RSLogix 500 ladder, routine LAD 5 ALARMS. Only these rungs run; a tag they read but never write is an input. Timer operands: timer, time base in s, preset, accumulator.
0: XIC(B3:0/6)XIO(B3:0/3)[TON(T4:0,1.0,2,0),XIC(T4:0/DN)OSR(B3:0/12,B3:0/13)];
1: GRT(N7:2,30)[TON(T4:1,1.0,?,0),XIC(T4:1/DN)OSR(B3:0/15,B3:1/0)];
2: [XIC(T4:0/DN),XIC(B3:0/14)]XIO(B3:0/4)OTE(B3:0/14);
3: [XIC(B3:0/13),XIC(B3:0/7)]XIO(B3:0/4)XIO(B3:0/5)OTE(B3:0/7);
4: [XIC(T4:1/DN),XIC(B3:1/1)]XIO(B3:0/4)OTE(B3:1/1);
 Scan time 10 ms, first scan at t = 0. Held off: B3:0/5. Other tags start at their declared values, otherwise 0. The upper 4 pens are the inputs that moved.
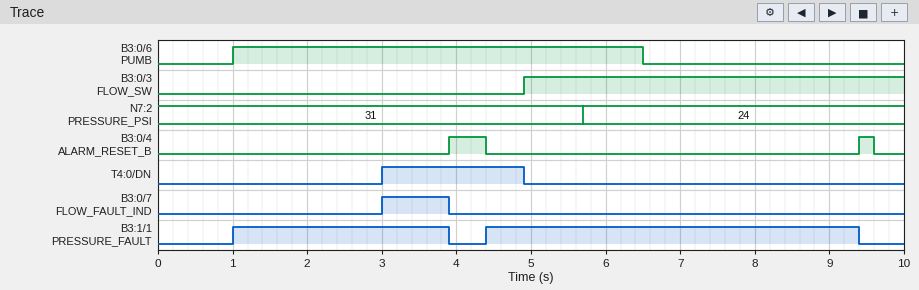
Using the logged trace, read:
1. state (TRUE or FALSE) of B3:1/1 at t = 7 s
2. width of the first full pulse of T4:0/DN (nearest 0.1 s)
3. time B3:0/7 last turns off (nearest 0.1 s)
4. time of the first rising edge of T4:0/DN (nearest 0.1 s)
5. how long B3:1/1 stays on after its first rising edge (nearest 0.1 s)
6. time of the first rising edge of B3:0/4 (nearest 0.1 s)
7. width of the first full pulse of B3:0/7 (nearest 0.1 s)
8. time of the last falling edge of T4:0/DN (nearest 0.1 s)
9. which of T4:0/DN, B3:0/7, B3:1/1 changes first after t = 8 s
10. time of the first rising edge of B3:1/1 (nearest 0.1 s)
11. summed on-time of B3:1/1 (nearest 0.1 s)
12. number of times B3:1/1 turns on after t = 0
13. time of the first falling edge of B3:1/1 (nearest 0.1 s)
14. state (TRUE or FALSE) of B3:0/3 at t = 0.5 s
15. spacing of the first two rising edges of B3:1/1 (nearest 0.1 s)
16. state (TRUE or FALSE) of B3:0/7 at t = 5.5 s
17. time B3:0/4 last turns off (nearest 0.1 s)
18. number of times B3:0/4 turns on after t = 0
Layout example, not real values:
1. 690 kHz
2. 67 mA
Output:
1. TRUE
2. 1.9 s
3. 3.9 s
4. 3.0 s
5. 2.9 s
6. 3.9 s
7. 0.9 s
8. 4.9 s
9. B3:1/1
10. 1.0 s
11. 7.9 s
12. 2
13. 3.9 s
14. FALSE
15. 3.4 s
16. FALSE
17. 9.6 s
18. 2
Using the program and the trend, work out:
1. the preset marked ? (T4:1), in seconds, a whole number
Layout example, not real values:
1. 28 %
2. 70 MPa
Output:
1. 1 s
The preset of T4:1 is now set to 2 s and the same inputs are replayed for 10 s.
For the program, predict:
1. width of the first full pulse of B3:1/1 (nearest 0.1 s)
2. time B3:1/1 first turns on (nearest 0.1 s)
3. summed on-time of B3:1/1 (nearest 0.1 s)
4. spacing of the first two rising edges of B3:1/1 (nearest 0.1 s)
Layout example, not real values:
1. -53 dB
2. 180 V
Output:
1. 1.9 s
2. 2.0 s
3. 6.9 s
4. 2.4 s
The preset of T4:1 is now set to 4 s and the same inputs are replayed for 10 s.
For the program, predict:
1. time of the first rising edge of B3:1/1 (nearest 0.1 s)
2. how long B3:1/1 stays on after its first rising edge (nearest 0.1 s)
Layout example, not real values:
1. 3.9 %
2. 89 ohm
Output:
1. 4.4 s
2. 5.0 s
